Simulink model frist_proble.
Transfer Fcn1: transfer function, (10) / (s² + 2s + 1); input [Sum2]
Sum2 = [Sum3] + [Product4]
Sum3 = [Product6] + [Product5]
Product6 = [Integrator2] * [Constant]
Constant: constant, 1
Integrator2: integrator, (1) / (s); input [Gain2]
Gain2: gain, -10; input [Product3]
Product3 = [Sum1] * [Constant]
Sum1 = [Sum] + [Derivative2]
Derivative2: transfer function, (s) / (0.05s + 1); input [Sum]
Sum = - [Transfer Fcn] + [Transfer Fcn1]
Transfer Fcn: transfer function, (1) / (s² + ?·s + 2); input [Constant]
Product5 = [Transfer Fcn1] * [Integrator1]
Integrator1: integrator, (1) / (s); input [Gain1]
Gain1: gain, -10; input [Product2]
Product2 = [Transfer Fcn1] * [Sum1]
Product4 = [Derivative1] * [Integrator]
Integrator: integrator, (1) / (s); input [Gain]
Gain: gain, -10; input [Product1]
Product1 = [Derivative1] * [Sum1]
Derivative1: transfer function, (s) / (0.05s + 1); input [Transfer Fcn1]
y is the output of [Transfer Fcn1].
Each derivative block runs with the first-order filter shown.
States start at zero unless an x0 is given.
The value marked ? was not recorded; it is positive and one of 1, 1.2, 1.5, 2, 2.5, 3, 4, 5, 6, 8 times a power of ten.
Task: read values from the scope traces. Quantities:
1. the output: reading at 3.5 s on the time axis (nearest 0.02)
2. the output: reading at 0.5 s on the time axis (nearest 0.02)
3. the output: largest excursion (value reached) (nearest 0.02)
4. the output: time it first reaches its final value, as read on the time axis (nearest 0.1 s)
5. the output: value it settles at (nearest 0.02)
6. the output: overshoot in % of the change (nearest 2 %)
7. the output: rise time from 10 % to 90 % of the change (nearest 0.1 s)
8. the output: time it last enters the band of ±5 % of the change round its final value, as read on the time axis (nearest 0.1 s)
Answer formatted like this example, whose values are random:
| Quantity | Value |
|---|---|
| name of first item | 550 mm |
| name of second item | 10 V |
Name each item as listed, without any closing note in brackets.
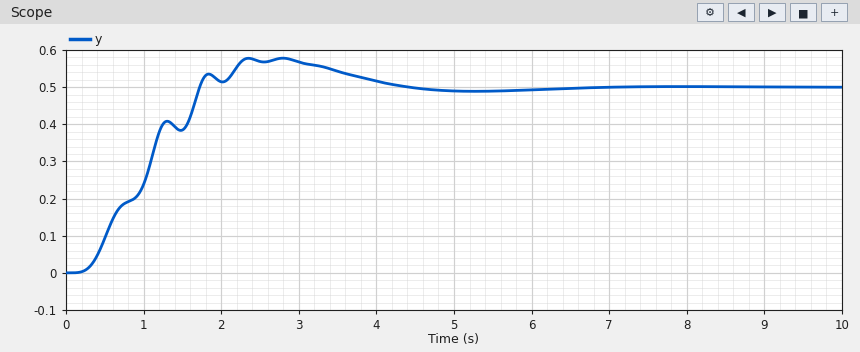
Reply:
| Quantity | Value |
|---|---|
| the output: reading at 3.5 s on the time axis | 0.54 |
| the output: reading at 0.5 s on the time axis | 0.10 |
| the output: largest excursion (value reached) | 0.58 |
| the output: time it first reaches its final value, as read on the time axis | 1.7 s |
| the output: value it settles at | 0.50 |
| the output: overshoot in % of the change | 16 % |
| the output: rise time from 10 % to 90 % of the change | 1.2 s |
| the output: time it last enters the band of ±5 % of the change round its final value, as read on the time axis | 3.8 s |
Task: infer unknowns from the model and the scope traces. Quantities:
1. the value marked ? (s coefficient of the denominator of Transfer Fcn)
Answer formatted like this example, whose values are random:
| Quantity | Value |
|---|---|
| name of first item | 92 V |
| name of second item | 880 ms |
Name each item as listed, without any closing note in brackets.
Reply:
| Quantity | Value |
|---|---|
| the value marked ? | 1.5 |
